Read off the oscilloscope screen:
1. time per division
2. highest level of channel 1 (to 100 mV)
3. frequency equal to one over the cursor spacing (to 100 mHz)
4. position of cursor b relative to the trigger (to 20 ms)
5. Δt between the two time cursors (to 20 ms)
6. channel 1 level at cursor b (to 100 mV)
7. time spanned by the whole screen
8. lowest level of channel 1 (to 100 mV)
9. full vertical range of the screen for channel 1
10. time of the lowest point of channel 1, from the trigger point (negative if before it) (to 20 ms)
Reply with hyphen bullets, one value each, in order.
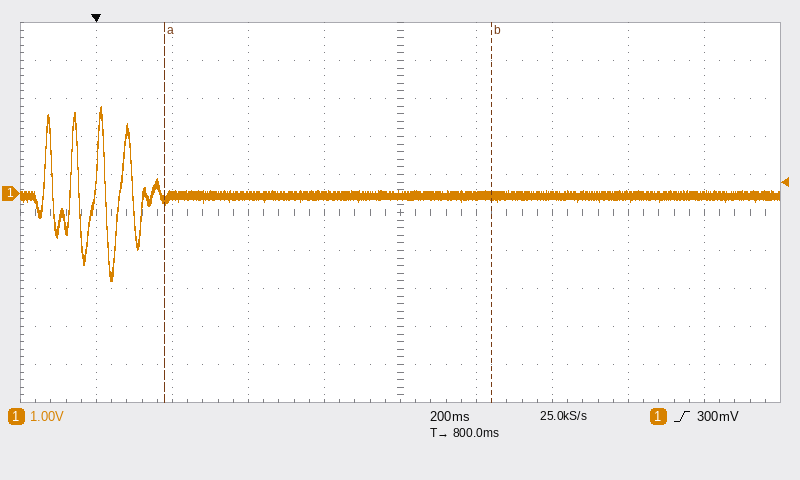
- 200 ms
- 2.3 V
- 1.2 Hz
- +1.04 s
- 860 ms
- -100 mV
- 2 s
- -2.3 V
- 10 V
- +40 ms
